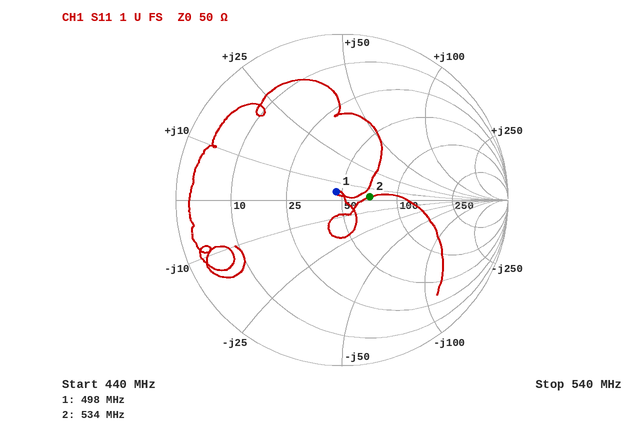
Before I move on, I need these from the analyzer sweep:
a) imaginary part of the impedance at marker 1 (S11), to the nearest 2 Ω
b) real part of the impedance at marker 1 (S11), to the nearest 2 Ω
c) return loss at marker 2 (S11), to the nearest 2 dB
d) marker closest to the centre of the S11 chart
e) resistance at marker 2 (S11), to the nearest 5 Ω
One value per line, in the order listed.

+4 Ω
46 Ω
16 dB
marker 1
70 Ω
